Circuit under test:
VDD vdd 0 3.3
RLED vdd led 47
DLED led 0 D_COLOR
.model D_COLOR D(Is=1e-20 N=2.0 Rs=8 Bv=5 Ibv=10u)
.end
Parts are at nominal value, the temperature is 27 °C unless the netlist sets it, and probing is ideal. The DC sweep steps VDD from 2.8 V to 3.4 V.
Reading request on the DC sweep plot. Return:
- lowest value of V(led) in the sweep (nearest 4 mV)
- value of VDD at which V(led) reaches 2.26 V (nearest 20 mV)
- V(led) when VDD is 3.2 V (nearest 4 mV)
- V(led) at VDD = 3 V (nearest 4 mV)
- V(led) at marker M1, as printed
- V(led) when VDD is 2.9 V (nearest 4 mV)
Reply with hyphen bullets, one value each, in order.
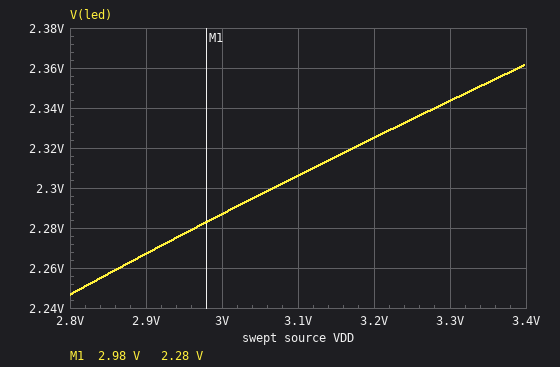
- 2.248 V
- 2.86 V
- 2.324 V
- 2.288 V
- 2.28 V
- 2.268 V
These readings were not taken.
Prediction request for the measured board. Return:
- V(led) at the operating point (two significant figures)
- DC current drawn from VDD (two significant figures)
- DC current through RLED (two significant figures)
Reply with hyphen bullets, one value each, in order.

- 2.3 V
- 20 mA
- 20 mA
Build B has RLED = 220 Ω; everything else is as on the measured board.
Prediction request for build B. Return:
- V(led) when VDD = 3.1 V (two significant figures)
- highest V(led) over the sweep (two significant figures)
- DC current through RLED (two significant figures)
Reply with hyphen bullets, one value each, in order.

- 2.1 V
- 2.2 V
- 5.2 mA
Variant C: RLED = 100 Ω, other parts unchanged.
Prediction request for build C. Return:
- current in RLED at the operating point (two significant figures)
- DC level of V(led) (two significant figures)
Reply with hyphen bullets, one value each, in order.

- 11 mA
- 2.2 V
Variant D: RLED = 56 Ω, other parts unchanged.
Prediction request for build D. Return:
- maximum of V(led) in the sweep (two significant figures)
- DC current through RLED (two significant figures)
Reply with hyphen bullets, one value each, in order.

- 2.3 V
- 18 mA
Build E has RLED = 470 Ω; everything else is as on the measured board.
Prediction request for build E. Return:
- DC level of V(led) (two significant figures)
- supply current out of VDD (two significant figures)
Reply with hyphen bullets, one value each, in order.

- 2.1 V
- 2.6 mA
